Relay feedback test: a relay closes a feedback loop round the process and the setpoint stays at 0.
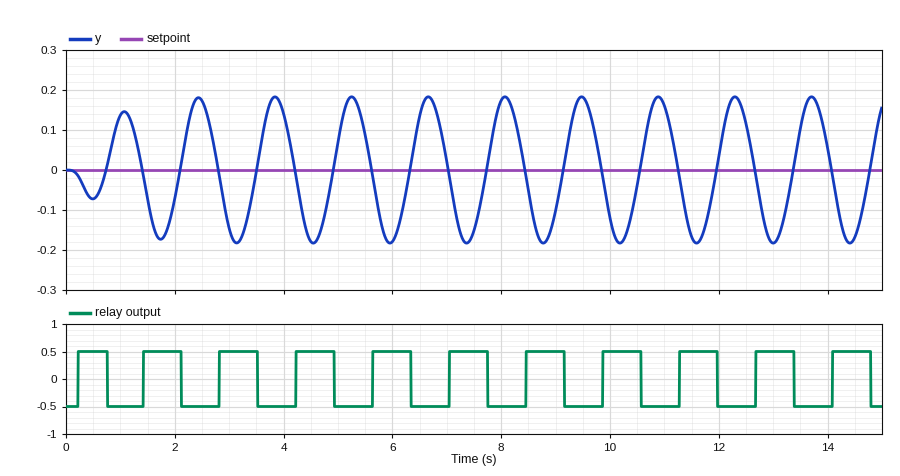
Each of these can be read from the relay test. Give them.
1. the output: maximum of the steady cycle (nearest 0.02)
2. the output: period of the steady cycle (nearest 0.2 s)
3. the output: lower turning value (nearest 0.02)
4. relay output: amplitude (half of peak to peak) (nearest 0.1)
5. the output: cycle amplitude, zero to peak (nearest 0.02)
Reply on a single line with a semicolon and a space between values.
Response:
0.18; 1.4 s; -0.18; 0.5; 0.18
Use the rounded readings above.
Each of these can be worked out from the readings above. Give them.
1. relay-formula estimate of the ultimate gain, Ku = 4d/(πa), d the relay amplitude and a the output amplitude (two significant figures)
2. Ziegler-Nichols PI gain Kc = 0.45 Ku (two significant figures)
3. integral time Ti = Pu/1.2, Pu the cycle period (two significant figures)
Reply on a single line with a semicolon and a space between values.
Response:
3.5; 1.6; 1.2 s
